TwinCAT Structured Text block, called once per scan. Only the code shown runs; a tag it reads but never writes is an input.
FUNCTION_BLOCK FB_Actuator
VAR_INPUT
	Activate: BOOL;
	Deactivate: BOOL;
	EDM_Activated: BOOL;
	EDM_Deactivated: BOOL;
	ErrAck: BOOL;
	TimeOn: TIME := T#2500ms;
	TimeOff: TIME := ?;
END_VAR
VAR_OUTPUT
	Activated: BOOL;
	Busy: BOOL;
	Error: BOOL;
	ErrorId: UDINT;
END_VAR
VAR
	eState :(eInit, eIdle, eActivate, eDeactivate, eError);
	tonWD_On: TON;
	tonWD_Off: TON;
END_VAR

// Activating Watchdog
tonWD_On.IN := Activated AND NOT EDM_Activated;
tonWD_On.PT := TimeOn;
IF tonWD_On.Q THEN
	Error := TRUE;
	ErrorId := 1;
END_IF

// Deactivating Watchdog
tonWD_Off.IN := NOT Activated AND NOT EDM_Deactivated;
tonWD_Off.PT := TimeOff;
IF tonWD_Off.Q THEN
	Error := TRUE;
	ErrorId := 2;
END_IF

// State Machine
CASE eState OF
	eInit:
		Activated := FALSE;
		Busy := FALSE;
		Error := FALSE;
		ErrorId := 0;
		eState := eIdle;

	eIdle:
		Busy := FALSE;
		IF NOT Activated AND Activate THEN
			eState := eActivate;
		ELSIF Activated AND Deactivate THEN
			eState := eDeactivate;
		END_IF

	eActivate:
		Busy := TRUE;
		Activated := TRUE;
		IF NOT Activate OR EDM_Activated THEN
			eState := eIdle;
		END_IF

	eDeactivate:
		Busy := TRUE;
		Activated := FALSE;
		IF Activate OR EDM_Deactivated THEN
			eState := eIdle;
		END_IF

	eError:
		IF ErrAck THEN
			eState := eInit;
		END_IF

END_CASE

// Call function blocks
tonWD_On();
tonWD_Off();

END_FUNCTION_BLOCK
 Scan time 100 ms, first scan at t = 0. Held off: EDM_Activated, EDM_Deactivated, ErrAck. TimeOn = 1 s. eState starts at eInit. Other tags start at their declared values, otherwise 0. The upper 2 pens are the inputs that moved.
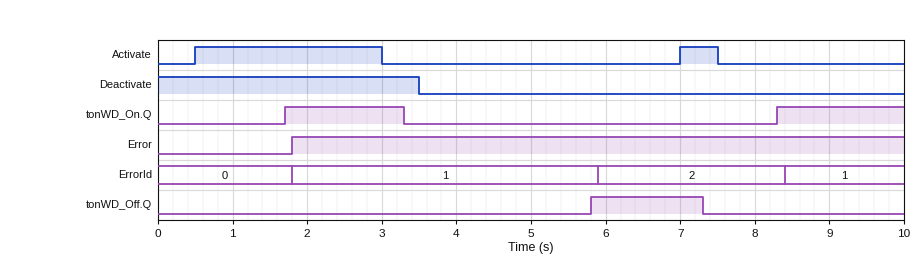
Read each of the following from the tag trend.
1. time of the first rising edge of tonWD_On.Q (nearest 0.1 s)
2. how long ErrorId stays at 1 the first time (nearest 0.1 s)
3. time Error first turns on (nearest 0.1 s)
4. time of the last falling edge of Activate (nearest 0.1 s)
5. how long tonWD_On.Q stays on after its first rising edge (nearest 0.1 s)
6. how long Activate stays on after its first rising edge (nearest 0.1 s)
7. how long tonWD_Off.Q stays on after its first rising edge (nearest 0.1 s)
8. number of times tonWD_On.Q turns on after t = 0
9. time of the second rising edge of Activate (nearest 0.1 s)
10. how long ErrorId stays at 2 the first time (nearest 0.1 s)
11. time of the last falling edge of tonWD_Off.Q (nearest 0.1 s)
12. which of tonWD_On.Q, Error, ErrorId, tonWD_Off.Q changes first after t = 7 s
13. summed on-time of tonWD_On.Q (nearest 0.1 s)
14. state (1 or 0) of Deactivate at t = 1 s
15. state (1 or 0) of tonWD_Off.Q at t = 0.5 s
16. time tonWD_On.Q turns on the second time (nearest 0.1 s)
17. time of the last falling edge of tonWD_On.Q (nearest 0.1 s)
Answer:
1.7 s
4.1 s
1.8 s
7.5 s
1.6 s
2.5 s
1.5 s
2
7.0 s
2.5 s
7.3 s
tonWD_Off.Q
3.3 s
1
0
8.3 s
3.3 s
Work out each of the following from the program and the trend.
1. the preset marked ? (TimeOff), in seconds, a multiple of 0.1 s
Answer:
2.5 s
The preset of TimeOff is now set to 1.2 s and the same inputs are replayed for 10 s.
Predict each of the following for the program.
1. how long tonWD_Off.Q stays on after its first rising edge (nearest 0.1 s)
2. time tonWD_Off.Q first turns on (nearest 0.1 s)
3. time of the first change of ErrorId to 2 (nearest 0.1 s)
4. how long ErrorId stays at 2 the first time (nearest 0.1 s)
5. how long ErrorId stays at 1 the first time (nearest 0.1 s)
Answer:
2.8 s
4.5 s
4.6 s
3.8 s
2.8 s
